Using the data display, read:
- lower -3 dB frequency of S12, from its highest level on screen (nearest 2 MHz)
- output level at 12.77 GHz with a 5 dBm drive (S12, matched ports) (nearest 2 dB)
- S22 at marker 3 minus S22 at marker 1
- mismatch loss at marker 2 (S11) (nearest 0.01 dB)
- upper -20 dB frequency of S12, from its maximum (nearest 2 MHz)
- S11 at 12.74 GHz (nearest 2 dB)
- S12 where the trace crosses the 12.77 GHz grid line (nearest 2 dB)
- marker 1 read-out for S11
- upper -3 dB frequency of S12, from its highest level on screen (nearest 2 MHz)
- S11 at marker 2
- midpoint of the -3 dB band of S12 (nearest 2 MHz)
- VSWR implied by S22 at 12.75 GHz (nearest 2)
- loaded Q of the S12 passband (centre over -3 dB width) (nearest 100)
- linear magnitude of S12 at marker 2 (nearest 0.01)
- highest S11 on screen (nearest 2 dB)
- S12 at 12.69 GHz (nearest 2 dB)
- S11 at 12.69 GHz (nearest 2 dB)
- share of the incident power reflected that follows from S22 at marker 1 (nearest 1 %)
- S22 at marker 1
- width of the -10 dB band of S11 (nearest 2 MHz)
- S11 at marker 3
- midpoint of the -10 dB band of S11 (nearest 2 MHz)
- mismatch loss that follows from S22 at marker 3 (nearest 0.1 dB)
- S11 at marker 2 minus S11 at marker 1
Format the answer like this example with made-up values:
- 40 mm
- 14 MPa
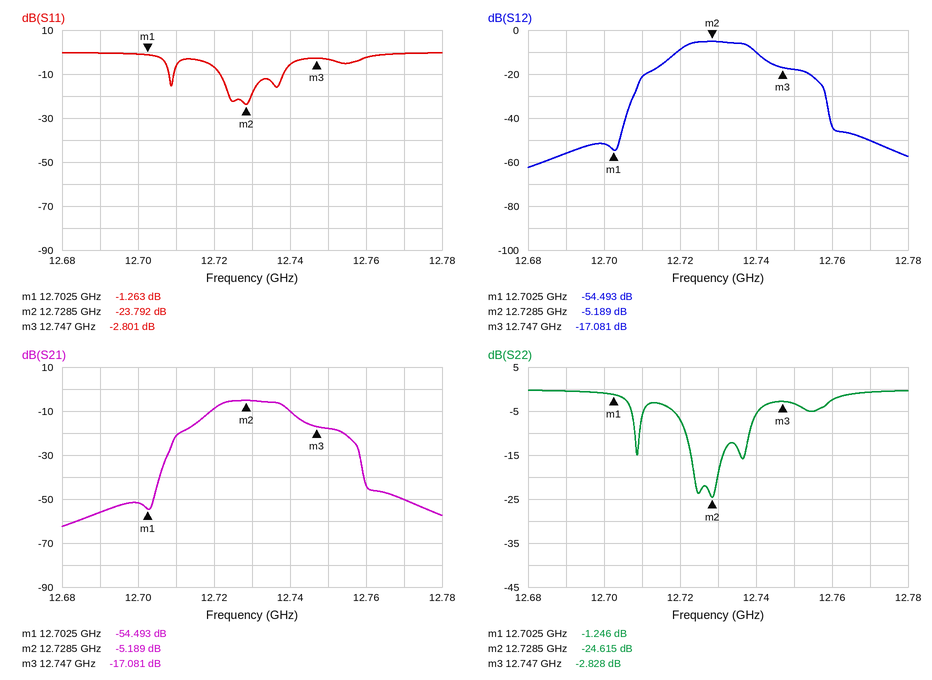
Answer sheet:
- 12.720 GHz
- -46 dBm
- -1.582 dB
- 0.02 dB
- 12.758 GHz
- -6 dB
- -50 dB
- -1.263 dB
- 12.738 GHz
- -23.792 dB
- 12.730 GHz
- 6
- 700
- 0.55
- 0 dB
- -56 dB
- 0 dB
- 75 %
- -1.246 dB
- 16 MHz
- -2.801 dB
- 12.730 GHz
- 3.2 dB
- -22.529 dB
